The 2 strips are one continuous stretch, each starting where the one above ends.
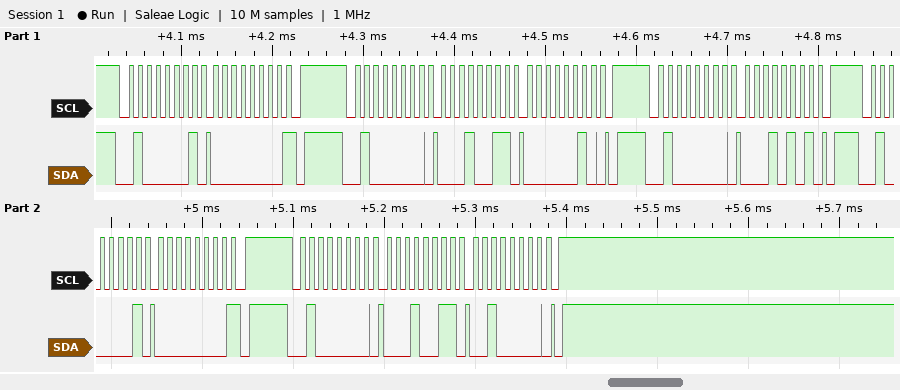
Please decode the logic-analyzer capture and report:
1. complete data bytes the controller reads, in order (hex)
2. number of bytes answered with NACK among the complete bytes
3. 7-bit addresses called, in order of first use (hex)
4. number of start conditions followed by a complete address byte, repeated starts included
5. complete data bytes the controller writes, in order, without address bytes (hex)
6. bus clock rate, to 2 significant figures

00 00
2
0x20
5
13 02 15 13 20
100 kHz
